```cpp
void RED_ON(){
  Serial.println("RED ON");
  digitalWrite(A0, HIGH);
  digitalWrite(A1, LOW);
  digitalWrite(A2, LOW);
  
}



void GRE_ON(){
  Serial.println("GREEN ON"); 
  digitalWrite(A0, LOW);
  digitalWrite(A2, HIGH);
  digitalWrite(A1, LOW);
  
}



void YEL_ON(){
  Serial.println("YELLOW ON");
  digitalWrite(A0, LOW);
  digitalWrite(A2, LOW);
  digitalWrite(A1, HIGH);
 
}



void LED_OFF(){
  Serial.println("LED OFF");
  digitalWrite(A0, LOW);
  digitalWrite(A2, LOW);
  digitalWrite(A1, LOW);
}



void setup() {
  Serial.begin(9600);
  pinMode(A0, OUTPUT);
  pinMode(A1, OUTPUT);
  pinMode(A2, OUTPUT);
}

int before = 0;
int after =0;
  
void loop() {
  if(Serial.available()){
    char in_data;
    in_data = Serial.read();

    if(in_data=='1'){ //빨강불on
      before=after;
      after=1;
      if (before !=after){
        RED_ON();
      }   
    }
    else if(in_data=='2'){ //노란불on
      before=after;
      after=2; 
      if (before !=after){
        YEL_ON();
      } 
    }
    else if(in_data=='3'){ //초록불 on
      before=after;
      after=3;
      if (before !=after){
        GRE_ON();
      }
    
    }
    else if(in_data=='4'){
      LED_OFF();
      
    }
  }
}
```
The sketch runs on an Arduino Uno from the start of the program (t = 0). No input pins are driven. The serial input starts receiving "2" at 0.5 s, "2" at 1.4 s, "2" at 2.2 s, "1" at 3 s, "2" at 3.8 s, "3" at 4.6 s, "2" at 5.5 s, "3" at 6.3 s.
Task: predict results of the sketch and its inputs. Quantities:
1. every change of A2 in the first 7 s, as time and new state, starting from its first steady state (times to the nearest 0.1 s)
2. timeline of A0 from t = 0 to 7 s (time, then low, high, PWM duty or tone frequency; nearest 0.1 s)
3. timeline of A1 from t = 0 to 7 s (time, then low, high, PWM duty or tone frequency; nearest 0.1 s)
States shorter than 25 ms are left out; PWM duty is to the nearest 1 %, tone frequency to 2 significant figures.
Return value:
0 s low; 4.6 s high; 5.5 s low; 6.3 s high
0 s low; 3 s high; 3.8 s low
0 s low; 0.5 s high; 3 s low; 3.8 s high; 4.6 s low; 5.5 s high; 6.3 s low
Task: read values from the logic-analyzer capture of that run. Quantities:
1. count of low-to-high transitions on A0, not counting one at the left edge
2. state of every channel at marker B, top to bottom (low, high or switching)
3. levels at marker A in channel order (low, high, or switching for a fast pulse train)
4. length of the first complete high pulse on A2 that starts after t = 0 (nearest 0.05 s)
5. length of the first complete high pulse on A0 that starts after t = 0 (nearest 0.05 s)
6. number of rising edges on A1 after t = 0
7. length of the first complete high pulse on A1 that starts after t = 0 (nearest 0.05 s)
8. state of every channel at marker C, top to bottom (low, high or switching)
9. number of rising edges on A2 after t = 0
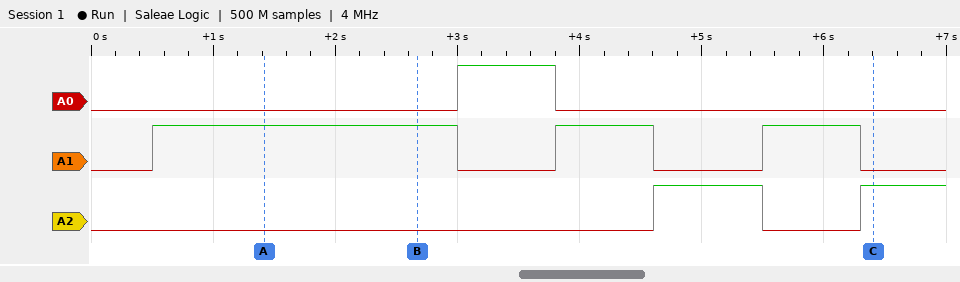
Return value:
1
A0 low, A1 high, A2 low
A0 low, A1 high, A2 low
0.90 s
0.80 s
3
2.50 s
A0 low, A1 low, A2 high
2
